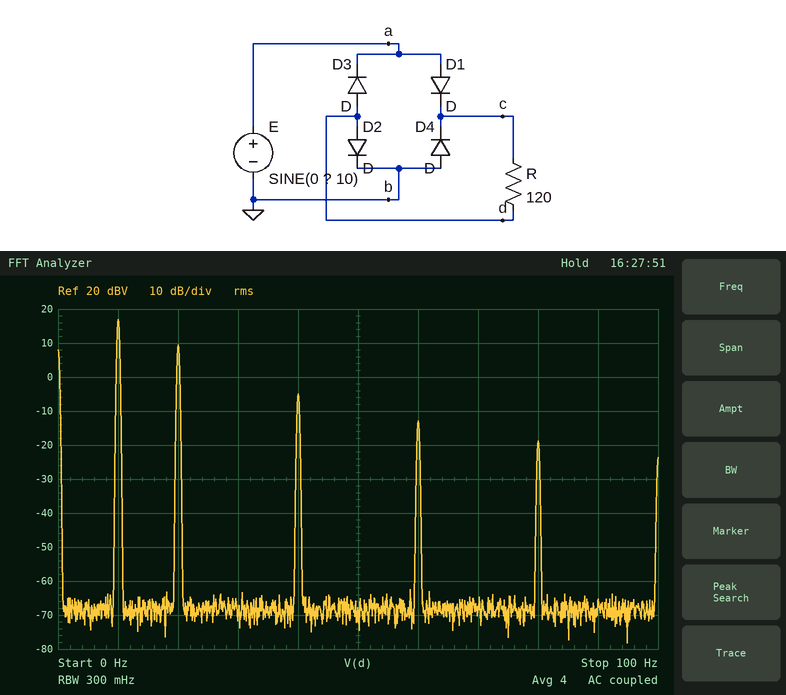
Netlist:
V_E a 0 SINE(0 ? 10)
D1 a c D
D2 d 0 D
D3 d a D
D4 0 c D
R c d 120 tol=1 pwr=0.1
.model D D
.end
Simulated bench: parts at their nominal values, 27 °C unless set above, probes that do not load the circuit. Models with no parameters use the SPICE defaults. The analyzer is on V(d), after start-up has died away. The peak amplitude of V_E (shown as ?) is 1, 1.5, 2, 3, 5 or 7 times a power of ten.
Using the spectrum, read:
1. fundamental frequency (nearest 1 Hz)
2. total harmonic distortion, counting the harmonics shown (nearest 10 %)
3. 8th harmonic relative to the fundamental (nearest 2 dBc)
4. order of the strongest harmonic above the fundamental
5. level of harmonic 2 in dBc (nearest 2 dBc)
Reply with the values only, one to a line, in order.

10 Hz
40 %
-36 dBc
2
-8 dBc
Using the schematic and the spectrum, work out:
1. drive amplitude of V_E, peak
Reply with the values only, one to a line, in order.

20 V
